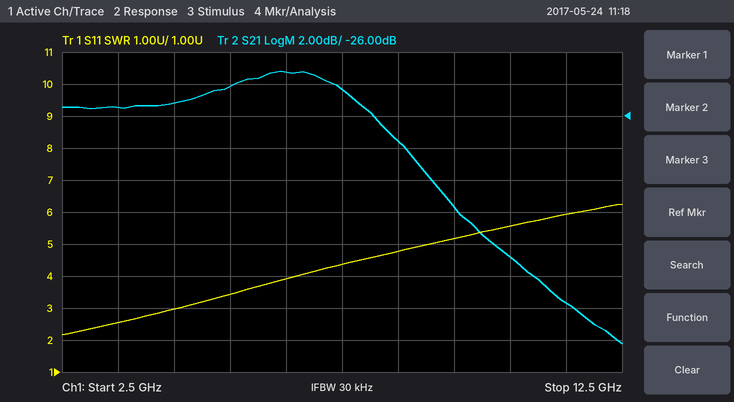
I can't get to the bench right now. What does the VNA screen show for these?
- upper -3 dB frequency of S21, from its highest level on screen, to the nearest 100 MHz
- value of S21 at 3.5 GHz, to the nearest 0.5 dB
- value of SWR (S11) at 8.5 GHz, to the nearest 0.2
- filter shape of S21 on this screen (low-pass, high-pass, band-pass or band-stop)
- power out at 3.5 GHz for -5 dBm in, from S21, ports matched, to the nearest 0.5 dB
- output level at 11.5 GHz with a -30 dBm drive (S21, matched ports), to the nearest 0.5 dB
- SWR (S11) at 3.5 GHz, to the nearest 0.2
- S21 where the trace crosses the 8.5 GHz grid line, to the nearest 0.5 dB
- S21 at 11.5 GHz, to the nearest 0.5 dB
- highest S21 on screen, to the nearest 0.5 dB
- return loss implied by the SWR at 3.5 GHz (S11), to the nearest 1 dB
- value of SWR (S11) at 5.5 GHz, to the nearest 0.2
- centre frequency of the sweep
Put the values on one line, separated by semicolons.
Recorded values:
8.1 GHz; -25.5 dB; 4.8; low-pass; -30.5 dBm; -67.5 dBm; 2.6; -27.5 dB; -37.5 dB; -23.0 dB; 7 dB; 3.4; 7.5 GHz
